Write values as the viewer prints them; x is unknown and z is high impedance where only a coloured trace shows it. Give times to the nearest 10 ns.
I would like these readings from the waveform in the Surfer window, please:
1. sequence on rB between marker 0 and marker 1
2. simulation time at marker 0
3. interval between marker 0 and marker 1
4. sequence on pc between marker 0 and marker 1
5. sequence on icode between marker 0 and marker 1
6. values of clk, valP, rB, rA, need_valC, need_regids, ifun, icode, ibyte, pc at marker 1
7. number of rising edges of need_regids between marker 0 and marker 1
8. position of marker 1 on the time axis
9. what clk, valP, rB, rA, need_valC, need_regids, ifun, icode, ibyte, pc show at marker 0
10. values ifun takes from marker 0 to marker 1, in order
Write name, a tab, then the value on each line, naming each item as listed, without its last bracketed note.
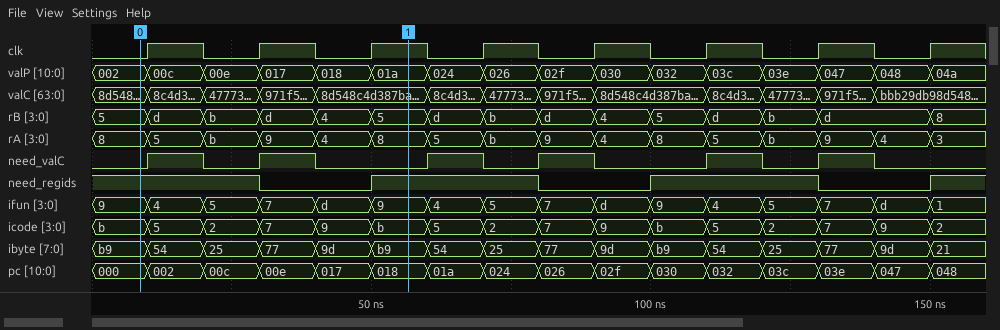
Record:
sequence on rB between marker 0 and marker 1	5, d, b, d, 4, 5
simulation time at marker 0	10 ns
interval between marker 0 and marker 1	50 ns
sequence on pc between marker 0 and marker 1	000, 002, 00c, 00e, 017, 018
sequence on icode between marker 0 and marker 1	b, 5, 2, 7, 9, b
values of clk, valP, rB, rA, need_valC, need_regids, ifun, icode, ibyte, pc at marker 1	clk=1, valP=01a, rB=5, rA=8, need_valC=0, need_regids=1, ifun=9, icode=b, ibyte=b9, pc=018
number of rising edges of need_regids between marker 0 and marker 1	1
position of marker 1 on the time axis	60 ns
what clk, valP, rB, rA, need_valC, need_regids, ifun, icode, ibyte, pc show at marker 0	clk=0, valP=002, rB=5, rA=8, need_valC=0, need_regids=1, ifun=9, icode=b, ibyte=b9, pc=000
values ifun takes from marker 0 to marker 1, in order	9, 4, 5, 7, d, 9
